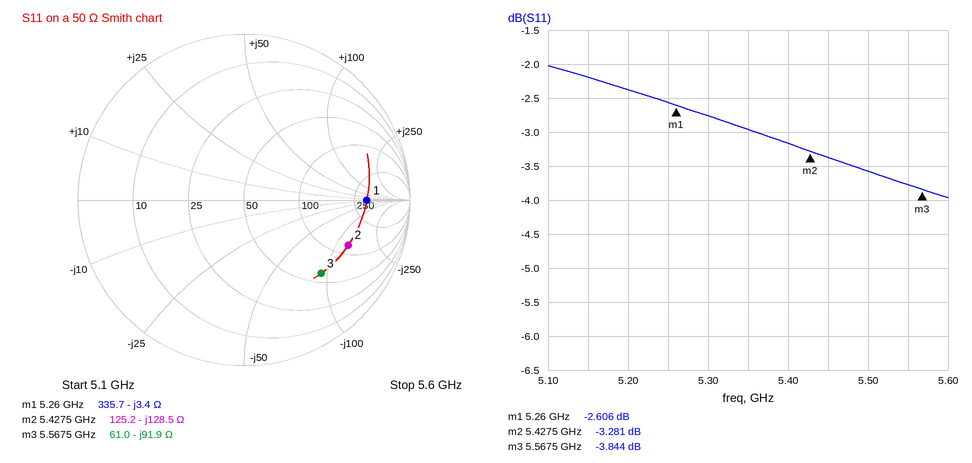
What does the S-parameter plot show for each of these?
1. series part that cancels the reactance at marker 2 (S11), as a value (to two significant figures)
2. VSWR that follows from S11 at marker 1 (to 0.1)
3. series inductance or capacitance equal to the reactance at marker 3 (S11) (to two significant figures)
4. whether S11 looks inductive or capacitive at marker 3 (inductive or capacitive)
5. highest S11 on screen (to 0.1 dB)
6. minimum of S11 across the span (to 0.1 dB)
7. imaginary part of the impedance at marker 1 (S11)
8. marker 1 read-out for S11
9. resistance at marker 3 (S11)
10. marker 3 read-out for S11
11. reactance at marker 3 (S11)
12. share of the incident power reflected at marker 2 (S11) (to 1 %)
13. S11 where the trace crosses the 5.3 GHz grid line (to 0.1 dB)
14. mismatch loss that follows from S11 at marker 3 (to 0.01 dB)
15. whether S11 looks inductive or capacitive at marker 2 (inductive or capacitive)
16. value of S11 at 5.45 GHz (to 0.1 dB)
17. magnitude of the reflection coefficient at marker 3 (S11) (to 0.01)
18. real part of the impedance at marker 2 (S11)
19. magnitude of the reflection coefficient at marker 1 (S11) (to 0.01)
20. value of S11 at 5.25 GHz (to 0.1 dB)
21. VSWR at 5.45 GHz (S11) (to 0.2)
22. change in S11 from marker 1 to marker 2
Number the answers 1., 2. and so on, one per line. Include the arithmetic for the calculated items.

1. L = 128.5 Ω/(2π × 5.4275 GHz) ≈ 3.8 nH
2. (1 + 0.7408)/(1 − 0.7408) ≈ 6.7
3. C = 1/(2π × 5.5675 GHz × 91.9 Ω) ≈ 311 fF, so 310 fF to two significant figures
4. capacitive
5. -2.0 dB
6. -4.0 dB
7. -3.4 Ω
8. -2.606 dB
9. 61.0 Ω
10. -3.844 dB
11. -91.9 Ω
12. 10^(-3.281/10) ≈ 47 %
13. -2.8 dB
14. −10 log10(1 − 10^(-3.844/10)) ≈ 2.31 dB
15. capacitive
16. -3.4 dB
17. 0.64
18. 125.2 Ω
19. 0.74
20. -2.6 dB
21. |Γ| = 10^(-3.4/20) = 0.6761; VSWR = (1 + 0.6761)/(1 − 0.6761) ≈ 5.2
22. -3.281 − (-2.606) = -0.675 dB
